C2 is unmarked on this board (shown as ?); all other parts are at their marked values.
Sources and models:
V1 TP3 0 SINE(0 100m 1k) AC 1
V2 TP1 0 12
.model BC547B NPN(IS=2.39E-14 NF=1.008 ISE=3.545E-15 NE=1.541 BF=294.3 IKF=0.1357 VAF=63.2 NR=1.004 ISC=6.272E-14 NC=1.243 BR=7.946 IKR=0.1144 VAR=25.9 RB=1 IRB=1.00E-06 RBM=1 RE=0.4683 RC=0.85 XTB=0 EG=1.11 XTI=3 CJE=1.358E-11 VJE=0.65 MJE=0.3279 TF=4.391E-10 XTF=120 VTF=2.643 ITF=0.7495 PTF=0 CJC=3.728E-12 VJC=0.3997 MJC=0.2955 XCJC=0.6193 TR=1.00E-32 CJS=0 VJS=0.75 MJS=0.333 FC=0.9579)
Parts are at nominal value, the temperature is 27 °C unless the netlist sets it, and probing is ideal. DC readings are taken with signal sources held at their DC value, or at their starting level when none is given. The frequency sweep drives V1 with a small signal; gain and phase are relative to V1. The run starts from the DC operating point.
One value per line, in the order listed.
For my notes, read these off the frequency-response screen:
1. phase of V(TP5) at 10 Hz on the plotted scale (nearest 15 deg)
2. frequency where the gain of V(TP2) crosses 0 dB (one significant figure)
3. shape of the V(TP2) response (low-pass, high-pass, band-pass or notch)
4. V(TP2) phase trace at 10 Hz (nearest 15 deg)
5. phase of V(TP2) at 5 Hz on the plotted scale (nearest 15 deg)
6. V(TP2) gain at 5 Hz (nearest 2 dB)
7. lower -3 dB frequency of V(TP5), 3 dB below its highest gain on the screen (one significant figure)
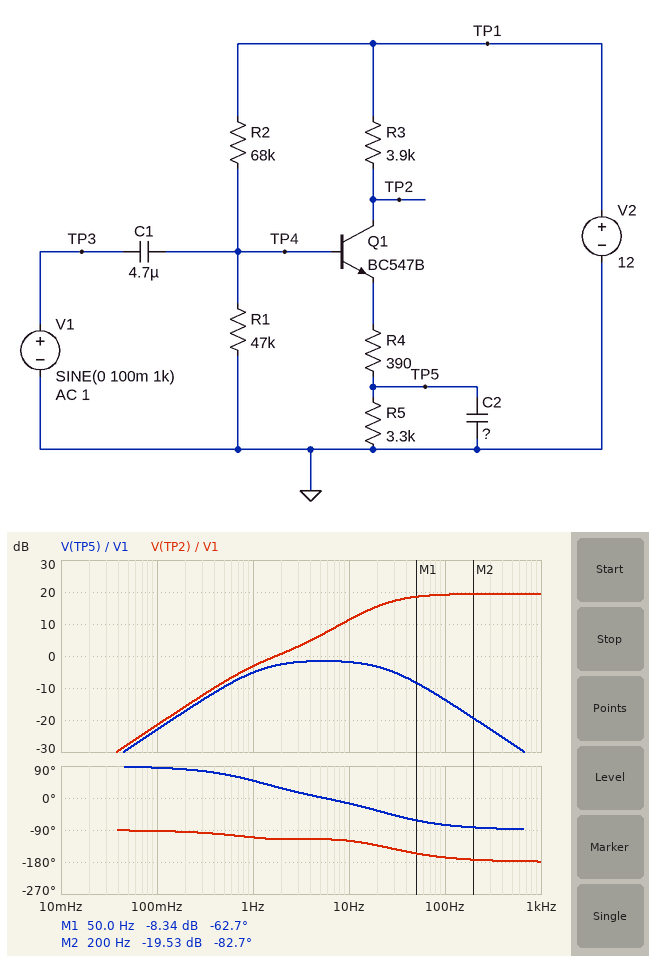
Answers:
-15 deg
2 Hz
high-pass
-120 deg
-120 deg
6 dB
1 Hz
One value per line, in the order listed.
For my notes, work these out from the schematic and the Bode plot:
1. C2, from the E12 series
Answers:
18 µF
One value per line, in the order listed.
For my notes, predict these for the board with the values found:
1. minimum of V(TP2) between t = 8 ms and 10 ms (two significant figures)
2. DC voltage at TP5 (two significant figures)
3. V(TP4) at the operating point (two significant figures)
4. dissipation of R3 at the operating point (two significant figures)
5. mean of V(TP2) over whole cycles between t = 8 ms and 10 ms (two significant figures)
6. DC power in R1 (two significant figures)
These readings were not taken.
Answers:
6.7 V
3.7 V
4.8 V
4.9 mW
7.6 V
490 µW
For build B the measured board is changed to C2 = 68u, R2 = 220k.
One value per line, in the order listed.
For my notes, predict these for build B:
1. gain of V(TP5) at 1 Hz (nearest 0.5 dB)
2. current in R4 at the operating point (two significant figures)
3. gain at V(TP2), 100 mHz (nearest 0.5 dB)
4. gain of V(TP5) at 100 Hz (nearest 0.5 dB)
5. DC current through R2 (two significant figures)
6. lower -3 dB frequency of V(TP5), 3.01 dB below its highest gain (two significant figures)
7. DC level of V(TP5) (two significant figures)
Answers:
-4.0 dB
390 µA
-19.0 dB
-26.0 dB
45 µA
690 mHz
1.3 V
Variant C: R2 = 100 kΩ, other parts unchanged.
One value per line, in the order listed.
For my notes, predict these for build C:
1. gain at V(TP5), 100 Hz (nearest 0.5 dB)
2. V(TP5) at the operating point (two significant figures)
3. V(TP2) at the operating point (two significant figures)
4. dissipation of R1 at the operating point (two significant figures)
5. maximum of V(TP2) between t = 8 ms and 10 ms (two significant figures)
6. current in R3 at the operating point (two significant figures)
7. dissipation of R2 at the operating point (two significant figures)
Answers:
-14.0 dB
2.8 V
8.7 V
300 µW
9.6 V
840 µA
680 µW
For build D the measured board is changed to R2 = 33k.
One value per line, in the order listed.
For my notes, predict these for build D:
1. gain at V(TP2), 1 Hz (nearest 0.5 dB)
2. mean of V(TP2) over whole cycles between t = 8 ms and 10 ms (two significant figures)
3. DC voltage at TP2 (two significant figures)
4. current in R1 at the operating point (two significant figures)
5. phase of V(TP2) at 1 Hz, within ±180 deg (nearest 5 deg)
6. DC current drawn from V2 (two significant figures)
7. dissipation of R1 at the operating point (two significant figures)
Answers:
-29.5 dB
6.3 V
5.9 V
140 µA
70 deg
1.7 mA
900 µW
